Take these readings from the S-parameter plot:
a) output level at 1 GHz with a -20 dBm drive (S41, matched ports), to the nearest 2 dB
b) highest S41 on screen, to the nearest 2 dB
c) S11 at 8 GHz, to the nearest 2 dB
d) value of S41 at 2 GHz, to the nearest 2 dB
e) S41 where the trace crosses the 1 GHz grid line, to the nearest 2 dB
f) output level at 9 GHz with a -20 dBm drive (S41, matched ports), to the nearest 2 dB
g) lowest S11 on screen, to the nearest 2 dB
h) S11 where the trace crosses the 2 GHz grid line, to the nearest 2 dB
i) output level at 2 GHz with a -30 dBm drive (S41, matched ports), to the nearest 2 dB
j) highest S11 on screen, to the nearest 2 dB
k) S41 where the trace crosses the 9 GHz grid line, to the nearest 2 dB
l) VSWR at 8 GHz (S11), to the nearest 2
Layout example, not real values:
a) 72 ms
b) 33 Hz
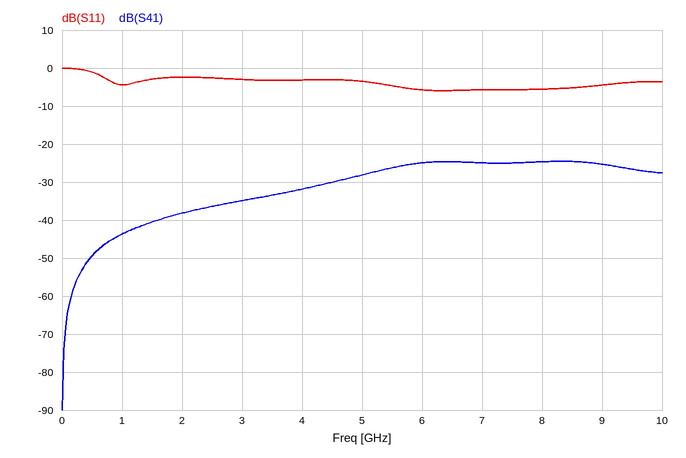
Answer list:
a) -64 dBm
b) -24 dB
c) -6 dB
d) -38 dB
e) -44 dB
f) -46 dBm
g) -6 dB
h) -2 dB
i) -68 dBm
j) 0 dB
k) -26 dB
l) 4
